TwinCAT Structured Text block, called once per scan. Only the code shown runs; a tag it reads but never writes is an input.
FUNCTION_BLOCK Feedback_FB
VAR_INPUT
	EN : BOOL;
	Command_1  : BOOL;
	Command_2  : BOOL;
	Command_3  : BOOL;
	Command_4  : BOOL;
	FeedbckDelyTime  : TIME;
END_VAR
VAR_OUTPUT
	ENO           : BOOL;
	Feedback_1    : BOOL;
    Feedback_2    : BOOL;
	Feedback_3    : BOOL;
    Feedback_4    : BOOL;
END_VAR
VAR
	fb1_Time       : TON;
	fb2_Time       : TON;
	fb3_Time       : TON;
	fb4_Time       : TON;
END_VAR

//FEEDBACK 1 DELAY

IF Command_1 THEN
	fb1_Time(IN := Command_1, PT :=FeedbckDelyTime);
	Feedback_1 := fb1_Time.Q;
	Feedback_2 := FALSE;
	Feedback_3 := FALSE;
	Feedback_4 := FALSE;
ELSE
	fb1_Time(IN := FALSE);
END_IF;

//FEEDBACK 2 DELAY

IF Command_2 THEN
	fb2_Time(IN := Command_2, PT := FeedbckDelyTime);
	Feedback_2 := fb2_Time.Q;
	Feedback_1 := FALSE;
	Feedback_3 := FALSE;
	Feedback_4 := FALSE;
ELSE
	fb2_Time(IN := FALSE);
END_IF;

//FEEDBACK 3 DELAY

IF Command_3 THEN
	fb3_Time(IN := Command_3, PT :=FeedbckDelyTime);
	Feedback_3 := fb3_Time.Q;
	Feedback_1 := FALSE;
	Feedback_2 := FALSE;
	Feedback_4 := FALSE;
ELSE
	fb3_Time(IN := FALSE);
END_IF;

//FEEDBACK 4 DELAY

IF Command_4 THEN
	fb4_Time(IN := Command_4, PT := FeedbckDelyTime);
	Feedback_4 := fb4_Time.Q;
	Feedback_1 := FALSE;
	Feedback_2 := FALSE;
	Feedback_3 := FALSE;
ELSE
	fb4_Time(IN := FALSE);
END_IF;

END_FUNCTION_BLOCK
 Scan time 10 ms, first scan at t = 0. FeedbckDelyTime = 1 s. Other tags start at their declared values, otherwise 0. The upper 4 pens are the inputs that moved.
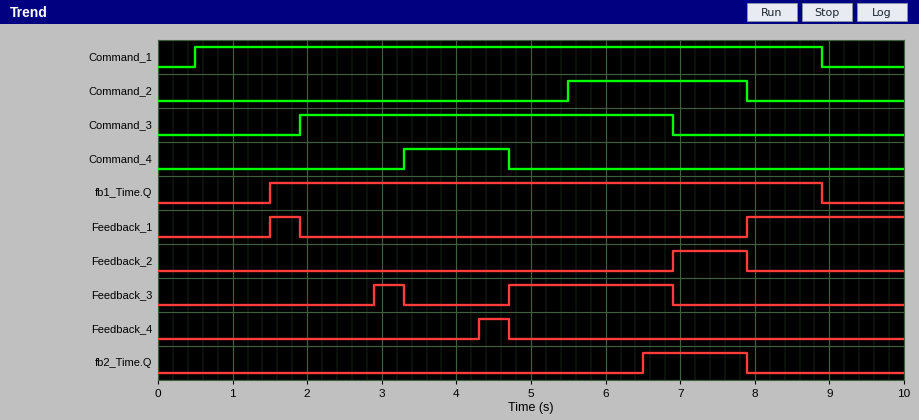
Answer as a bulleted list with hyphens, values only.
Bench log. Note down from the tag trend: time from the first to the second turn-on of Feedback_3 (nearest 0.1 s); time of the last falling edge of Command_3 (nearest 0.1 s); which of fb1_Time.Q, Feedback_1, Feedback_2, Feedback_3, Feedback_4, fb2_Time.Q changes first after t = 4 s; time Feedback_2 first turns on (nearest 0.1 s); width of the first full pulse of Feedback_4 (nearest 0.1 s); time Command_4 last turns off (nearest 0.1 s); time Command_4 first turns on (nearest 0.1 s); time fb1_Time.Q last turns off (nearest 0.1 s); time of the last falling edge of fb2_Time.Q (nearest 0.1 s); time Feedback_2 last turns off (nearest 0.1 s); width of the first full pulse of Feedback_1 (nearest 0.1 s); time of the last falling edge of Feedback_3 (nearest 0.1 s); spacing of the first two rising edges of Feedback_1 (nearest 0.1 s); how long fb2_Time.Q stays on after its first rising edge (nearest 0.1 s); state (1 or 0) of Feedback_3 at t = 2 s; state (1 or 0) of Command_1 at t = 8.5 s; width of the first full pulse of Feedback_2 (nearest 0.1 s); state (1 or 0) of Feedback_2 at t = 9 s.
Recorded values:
- 1.8 s
- 6.9 s
- Feedback_4
- 6.9 s
- 0.4 s
- 4.7 s
- 3.3 s
- 8.9 s
- 7.9 s
- 7.9 s
- 0.4 s
- 6.9 s
- 6.4 s
- 1.4 s
- 0
- 1
- 1.0 s
- 0
